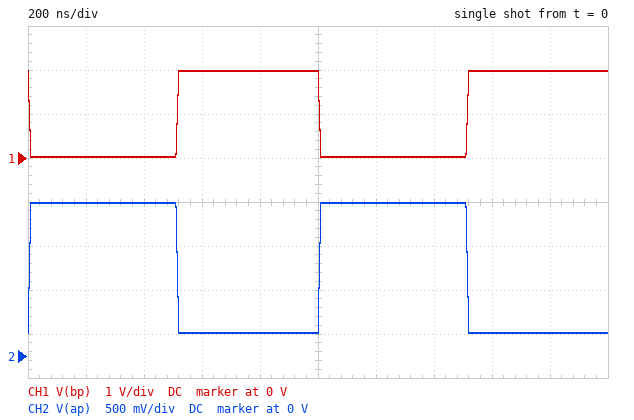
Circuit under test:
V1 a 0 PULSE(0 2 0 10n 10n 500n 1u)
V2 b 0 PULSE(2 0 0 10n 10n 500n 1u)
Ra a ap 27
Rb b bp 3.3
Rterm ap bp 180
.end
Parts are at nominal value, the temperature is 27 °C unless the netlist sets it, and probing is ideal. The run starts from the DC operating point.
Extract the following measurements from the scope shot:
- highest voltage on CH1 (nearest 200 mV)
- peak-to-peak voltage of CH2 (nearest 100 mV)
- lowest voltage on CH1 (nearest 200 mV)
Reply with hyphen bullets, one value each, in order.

- 2.0 V
- 1.5 V
- 0 V
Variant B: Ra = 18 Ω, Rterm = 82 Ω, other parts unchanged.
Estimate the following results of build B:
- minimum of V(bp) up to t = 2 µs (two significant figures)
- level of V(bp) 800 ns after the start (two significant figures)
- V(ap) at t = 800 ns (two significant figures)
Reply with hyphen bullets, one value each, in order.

- 64 mV
- 1.9 V
- 350 mV
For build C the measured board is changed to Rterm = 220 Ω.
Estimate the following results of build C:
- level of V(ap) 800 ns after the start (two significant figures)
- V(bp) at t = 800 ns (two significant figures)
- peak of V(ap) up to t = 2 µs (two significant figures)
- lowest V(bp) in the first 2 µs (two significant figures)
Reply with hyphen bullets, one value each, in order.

- 220 mV
- 2.0 V
- 1.8 V
- 26 mV
